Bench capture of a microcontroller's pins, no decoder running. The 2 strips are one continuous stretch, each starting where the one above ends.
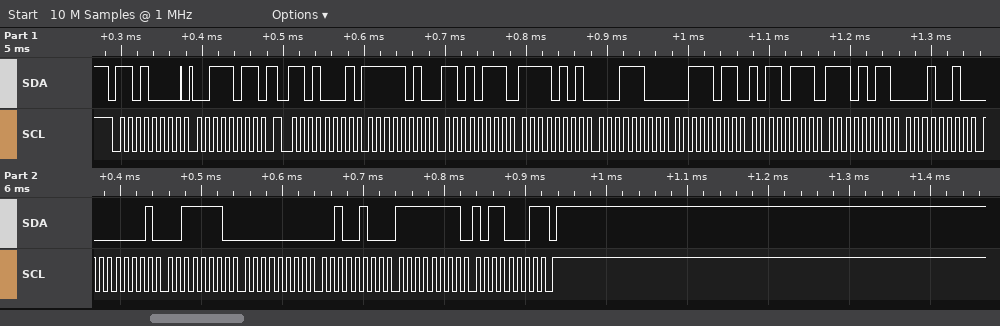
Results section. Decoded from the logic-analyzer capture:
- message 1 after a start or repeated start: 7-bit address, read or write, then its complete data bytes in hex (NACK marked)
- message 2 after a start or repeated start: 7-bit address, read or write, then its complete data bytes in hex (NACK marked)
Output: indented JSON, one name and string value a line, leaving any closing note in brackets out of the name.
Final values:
{
  "message 1 after a start or repeated start: 7-bit address, read or write, then its complete data bytes in hex": "0x68 write: 3B",
  "message 2 after a start or repeated start: 7-bit address, read or write, then its complete data bytes in hex": "0x68 read: FA D7 F5 1C 3B B7 EB 12 01 3E 00 24 FF B1 NACK"
}
